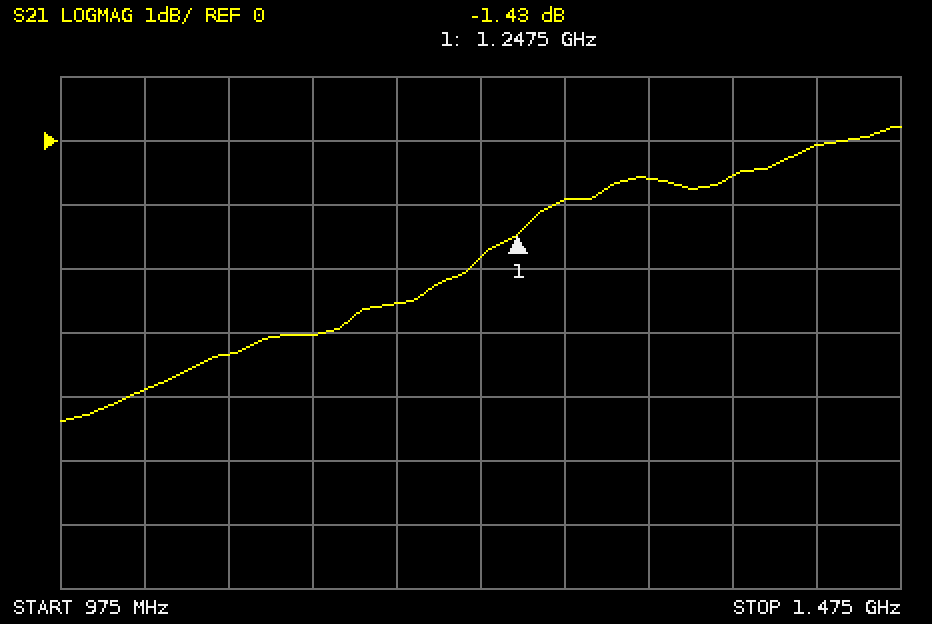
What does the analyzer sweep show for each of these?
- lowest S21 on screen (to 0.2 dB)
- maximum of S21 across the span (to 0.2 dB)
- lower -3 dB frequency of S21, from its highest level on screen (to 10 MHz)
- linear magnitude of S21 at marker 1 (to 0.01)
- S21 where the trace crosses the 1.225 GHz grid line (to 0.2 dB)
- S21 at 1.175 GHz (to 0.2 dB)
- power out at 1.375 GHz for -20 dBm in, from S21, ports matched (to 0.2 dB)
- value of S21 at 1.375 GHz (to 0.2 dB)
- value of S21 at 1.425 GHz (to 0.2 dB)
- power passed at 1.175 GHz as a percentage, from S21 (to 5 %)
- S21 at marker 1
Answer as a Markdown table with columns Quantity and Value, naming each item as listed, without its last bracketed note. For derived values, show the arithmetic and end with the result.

| Quantity | Value |
|---|---|
| lowest S21 on screen | -4.4 dB |
| maximum of S21 across the span | 0.2 dB |
| lower -3 dB frequency of S21, from its highest level on screen | 1.15 GHz |
| linear magnitude of S21 at marker 1 | 10^(-1.43/20) ≈ 0.85 |
| S21 where the trace crosses the 1.225 GHz grid line | -1.8 dB |
| S21 at 1.175 GHz | -2.6 dB |
| power out at 1.375 GHz for -20 dBm in, from S21, ports matched | -20 dBm + (-0.6 dB) = -20.6 dBm |
| value of S21 at 1.375 GHz | -0.6 dB |
| value of S21 at 1.425 GHz | 0.0 dB |
| power passed at 1.175 GHz as a percentage, from S21 | 10^(-2.6/10) ≈ 55 % |
| S21 at marker 1 | -1.43 dB |
